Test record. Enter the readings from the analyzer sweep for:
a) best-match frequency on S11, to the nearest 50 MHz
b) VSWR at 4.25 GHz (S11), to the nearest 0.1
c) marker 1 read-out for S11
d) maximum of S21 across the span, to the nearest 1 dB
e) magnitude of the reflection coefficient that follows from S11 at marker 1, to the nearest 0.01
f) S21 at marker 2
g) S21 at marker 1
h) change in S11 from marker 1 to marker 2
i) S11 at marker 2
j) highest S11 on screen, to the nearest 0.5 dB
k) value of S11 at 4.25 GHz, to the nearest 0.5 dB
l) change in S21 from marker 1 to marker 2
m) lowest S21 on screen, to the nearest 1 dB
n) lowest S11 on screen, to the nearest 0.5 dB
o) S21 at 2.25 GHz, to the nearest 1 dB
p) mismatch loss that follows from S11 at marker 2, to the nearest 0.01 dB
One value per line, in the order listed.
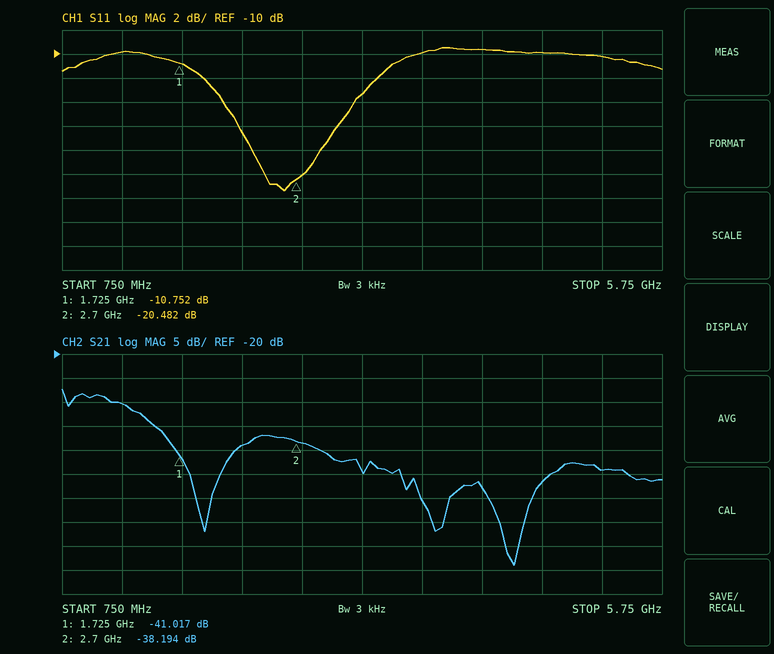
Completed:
2.60 GHz
2.0
-10.752 dB
-27 dB
0.29
-38.194 dB
-41.017 dB
-9.730 dB
-20.482 dB
-9.5 dB
-9.5 dB
2.823 dB
-64 dB
-21.5 dB
-39 dB
0.04 dB
